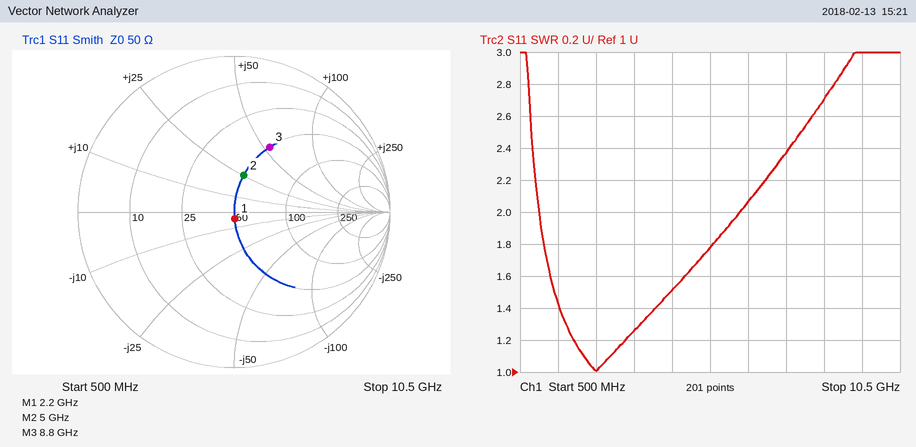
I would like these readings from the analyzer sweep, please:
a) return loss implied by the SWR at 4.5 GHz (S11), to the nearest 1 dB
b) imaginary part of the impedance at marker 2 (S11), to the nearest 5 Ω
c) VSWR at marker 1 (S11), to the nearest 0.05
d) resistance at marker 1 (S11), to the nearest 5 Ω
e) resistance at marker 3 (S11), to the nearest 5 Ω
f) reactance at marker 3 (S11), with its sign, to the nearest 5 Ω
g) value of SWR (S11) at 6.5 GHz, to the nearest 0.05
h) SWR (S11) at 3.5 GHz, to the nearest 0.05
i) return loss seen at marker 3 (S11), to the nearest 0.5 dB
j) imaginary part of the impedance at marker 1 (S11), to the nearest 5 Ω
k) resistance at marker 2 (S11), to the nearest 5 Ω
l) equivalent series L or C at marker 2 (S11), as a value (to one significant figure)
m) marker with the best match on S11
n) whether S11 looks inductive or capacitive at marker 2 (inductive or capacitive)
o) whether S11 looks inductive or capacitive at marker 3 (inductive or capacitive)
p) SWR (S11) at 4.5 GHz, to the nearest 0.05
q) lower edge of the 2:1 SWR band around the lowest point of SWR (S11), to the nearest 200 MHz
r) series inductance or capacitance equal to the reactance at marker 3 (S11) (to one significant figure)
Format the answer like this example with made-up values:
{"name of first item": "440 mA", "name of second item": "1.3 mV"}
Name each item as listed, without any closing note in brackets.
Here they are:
{"return loss implied by the SWR at 4.5 GHz (S11), to the nearest 1 dB": "14 dB", "imaginary part of the impedance at marker 2 (S11), to the nearest 5 Ω": "+25 Ω", "VSWR at marker 1 (S11), to the nearest 0.05": "1.10", "resistance at marker 1 (S11), to the nearest 5 Ω": "50 Ω", "resistance at marker 3 (S11), to the nearest 5 Ω": "50 Ω", "reactance at marker 3 (S11), with its sign, to the nearest 5 Ω": "+55 Ω", "value of SWR (S11) at 6.5 GHz, to the nearest 0.05": "2.05", "SWR (S11) at 3.5 GHz, to the nearest 0.05": "1.25", "return loss seen at marker 3 (S11), to the nearest 0.5 dB": "6.5 dB", "imaginary part of the impedance at marker 1 (S11), to the nearest 5 Ω": "-5 Ω", "resistance at marker 2 (S11), to the nearest 5 Ω": "50 Ω", "equivalent series L or C at marker 2 (S11), as a value": "800 pH", "marker with the best match on S11": "marker 1", "whether S11 looks inductive or capacitive at marker 2": "inductive", "whether S11 looks inductive or capacitive at marker 3": "inductive", "SWR (S11) at 4.5 GHz, to the nearest 0.05": "1.50", "lower edge of the 2:1 SWR band around the lowest point of SWR (S11), to the nearest 200 MHz": "1.0 GHz", "series inductance or capacitance equal to the reactance at marker 3 (S11)": "1.0 nH"}
